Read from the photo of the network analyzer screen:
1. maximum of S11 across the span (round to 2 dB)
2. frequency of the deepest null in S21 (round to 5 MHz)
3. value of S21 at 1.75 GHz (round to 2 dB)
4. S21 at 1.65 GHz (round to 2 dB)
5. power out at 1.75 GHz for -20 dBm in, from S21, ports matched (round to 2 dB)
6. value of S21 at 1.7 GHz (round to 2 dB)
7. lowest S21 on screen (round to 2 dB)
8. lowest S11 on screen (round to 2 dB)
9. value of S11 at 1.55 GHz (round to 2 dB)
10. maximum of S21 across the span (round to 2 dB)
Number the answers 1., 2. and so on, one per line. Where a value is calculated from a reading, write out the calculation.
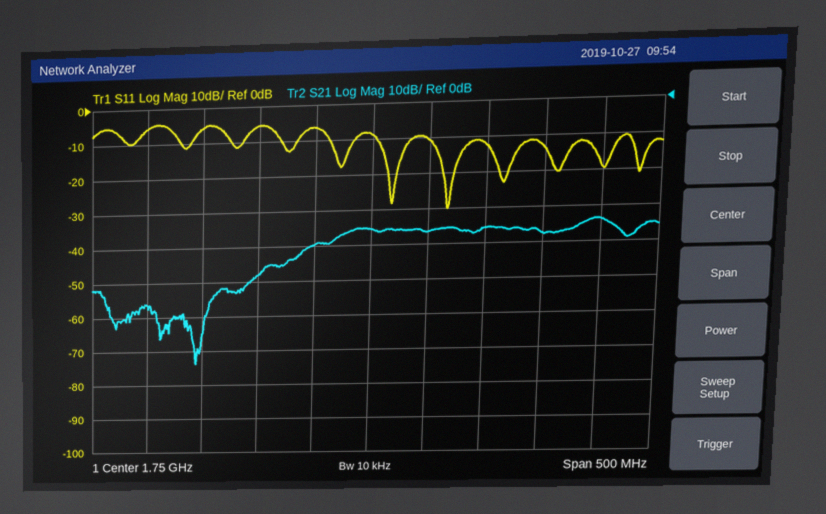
1. -4 dB
2. 1.595 GHz
3. -36 dB
4. -48 dB
5. -20 dBm + (-36 dB) = -56 dBm
6. -40 dB
7. -74 dB
8. -30 dB
9. -6 dB
10. -34 dB
